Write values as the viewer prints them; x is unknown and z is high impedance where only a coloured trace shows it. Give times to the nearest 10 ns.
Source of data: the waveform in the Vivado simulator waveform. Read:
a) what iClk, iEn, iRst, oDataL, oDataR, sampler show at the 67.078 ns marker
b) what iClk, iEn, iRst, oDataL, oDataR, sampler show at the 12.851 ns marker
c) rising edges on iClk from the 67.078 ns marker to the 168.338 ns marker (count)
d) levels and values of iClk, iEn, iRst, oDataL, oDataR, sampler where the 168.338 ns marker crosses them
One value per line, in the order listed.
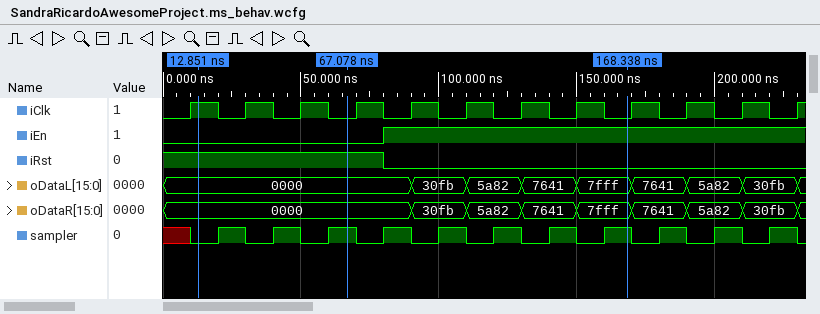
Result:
iClk=0, iEn=0, iRst=1, oDataL=0000, oDataR=0000, sampler=1
iClk=1, iEn=0, iRst=1, oDataL=0000, oDataR=0000, sampler=0
5
iClk=0, iEn=1, iRst=0, oDataL=7fff, oDataR=7fff, sampler=1
